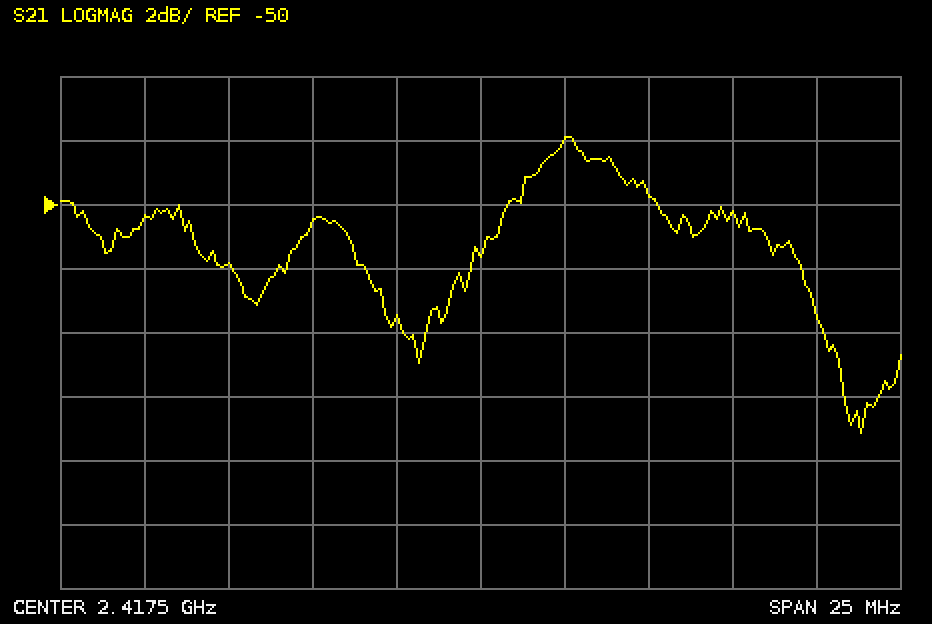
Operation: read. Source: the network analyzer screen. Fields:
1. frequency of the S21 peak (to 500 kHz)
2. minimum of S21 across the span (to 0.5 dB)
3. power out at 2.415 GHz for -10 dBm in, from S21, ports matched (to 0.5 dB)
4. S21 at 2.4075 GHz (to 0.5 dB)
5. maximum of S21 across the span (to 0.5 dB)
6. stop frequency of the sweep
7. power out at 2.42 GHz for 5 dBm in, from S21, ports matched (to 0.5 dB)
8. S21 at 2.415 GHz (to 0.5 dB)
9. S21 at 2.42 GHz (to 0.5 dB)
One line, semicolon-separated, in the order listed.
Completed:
2.4200 GHz; -57.0 dB; -63.5 dBm; -50.5 dB; -48.0 dB; 2.43 GHz; -43.0 dBm; -53.5 dB; -48.0 dB
